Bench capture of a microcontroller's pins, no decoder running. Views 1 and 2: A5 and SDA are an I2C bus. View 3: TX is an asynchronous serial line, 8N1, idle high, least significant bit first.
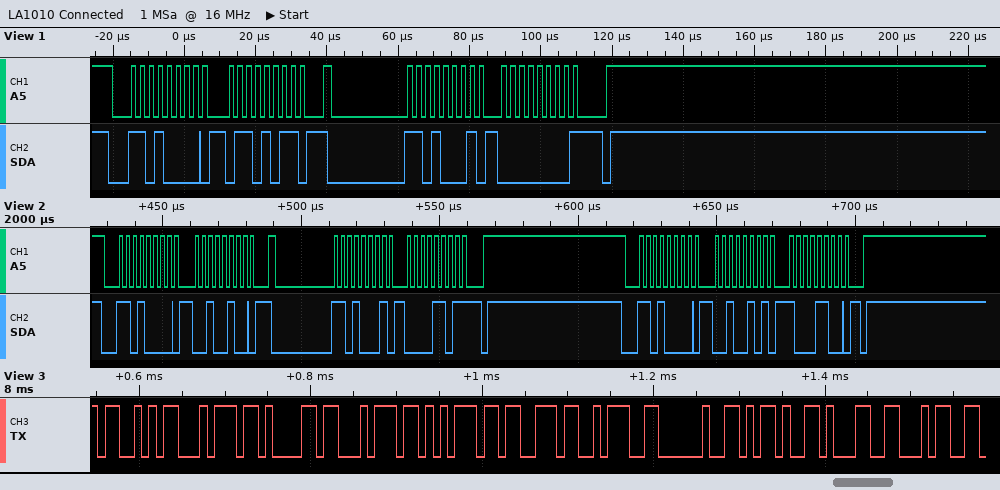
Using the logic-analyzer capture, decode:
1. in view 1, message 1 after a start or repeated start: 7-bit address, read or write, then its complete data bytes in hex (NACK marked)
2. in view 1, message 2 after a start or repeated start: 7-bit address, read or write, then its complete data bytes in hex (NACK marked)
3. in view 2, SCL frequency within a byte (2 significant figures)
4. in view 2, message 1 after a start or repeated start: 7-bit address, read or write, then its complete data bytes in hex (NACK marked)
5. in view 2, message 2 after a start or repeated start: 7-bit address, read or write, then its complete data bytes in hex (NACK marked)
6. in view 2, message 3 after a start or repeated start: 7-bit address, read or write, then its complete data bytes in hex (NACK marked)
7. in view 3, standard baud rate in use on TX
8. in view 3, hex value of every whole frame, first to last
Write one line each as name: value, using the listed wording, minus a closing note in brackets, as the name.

in view 1, message 1 after a start or repeated start: 7-bit address, read or write, then its complete data bytes in hex: 0x68 write: 6B
in view 1, message 2 after a start or repeated start: 7-bit address, read or write, then its complete data bytes in hex: 0x68 read: 00 NACK
in view 2, SCL frequency within a byte: 400 kHz
in view 2, message 1 after a start or repeated start: 7-bit address, read or write, then its complete data bytes in hex: 0x68 write: 24
in view 2, message 2 after a start or repeated start: 7-bit address, read or write, then its complete data bytes in hex: 0x68 read: 0D NACK
in view 2, message 3 after a start or repeated start: 7-bit address, read or write, then its complete data bytes in hex: 0x68 write: 25 8C
in view 3, standard baud rate in use on TX: 115200 baud
in view 3, hex value of every whole frame, first to last: 53 74 61 74 75 73 3A 20 2D 31 34
